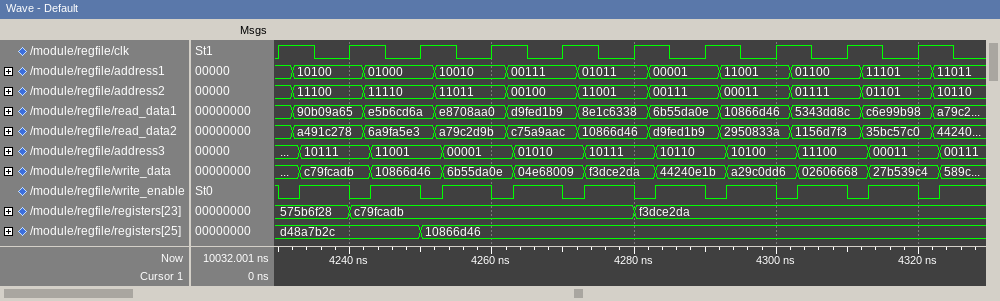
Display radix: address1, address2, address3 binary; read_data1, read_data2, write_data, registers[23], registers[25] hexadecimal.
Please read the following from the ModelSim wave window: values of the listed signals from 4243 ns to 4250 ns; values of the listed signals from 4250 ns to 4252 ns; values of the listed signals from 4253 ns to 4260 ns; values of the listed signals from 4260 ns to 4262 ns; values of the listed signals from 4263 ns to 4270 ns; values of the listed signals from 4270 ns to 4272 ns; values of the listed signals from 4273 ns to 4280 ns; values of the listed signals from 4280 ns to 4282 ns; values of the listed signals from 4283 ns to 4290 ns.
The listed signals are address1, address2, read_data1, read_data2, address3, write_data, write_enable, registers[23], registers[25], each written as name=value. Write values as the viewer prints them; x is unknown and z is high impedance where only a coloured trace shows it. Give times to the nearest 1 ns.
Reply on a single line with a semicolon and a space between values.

address1=01000, address2=11110, read_data1=e5b6cd6a, read_data2=6a9fa5e3, address3=11001, write_data=10866d46, write_enable=1, registers[23]=c79fcadb, registers[25]=d48a7b2c; address1=01000, address2=11110, read_data1=e5b6cd6a, read_data2=6a9fa5e3, address3=11001, write_data=10866d46, write_enable=0, registers[23]=c79fcadb, registers[25]=10866d46; address1=10010, address2=11011, read_data1=e8708aa0, read_data2=a79c2d9b, address3=00001, write_data=6b55da0e, write_enable=1, registers[23]=c79fcadb, registers[25]=10866d46; address1=10010, address2=11011, read_data1=e8708aa0, read_data2=a79c2d9b, address3=00001, write_data=6b55da0e, write_enable=0, registers[23]=c79fcadb, registers[25]=10866d46; address1=00111, address2=00100, read_data1=d9fed1b9, read_data2=c75a9aac, address3=01010, write_data=04e68009, write_enable=1, registers[23]=c79fcadb, registers[25]=10866d46; address1=00111, address2=00100, read_data1=d9fed1b9, read_data2=c75a9aac, address3=01010, write_data=04e68009, write_enable=0, registers[23]=c79fcadb, registers[25]=10866d46; address1=01011, address2=11001, read_data1=8e1c6338, read_data2=10866d46, address3=10111, write_data=f3dce2da, write_enable=1, registers[23]=c79fcadb, registers[25]=10866d46; address1=01011, address2=11001, read_data1=8e1c6338, read_data2=10866d46, address3=10111, write_data=f3dce2da, write_enable=0, registers[23]=f3dce2da, registers[25]=10866d46; address1=00001, address2=00111, read_data1=6b55da0e, read_data2=d9fed1b9, address3=10110, write_data=44240e1b, write_enable=1, registers[23]=f3dce2da, registers[25]=10866d46
